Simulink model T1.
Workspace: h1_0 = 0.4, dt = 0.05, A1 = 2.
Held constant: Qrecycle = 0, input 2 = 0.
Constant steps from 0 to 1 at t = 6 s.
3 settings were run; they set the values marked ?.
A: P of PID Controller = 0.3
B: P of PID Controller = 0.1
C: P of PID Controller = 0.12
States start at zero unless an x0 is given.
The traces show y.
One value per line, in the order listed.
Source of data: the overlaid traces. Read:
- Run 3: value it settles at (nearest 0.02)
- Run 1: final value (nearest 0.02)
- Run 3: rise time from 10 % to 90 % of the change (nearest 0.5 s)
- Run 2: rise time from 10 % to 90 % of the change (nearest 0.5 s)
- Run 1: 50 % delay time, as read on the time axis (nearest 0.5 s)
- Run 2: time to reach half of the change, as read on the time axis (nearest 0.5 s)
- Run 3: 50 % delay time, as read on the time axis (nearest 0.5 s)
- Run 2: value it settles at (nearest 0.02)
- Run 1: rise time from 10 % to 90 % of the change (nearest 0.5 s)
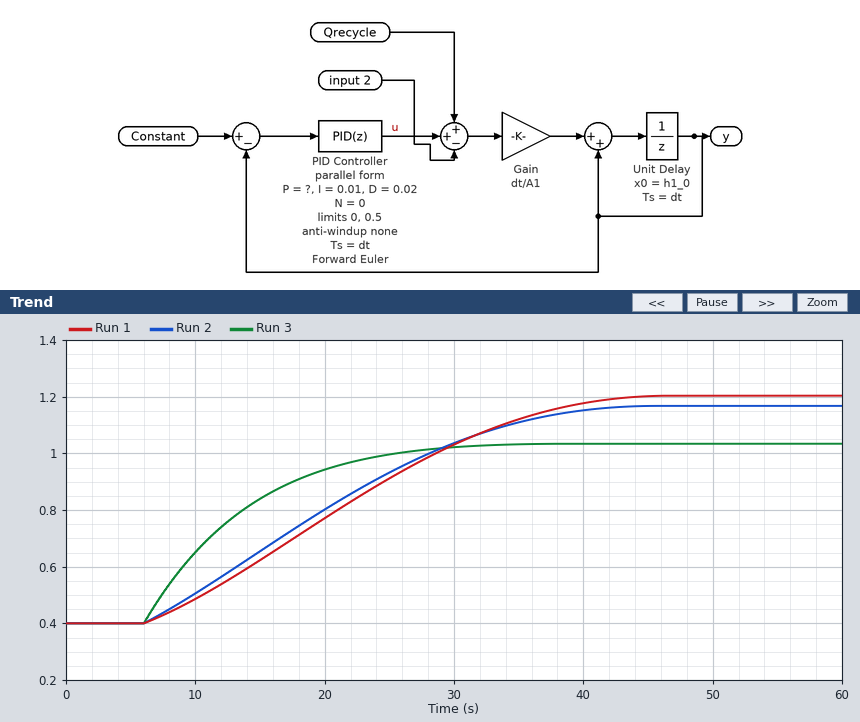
1.04
1.20
15.5 s
24.5 s
21.0 s
19.5 s
11.5 s
1.16
25.5 s
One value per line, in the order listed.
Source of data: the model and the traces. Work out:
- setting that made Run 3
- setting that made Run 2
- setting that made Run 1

A
C
B
